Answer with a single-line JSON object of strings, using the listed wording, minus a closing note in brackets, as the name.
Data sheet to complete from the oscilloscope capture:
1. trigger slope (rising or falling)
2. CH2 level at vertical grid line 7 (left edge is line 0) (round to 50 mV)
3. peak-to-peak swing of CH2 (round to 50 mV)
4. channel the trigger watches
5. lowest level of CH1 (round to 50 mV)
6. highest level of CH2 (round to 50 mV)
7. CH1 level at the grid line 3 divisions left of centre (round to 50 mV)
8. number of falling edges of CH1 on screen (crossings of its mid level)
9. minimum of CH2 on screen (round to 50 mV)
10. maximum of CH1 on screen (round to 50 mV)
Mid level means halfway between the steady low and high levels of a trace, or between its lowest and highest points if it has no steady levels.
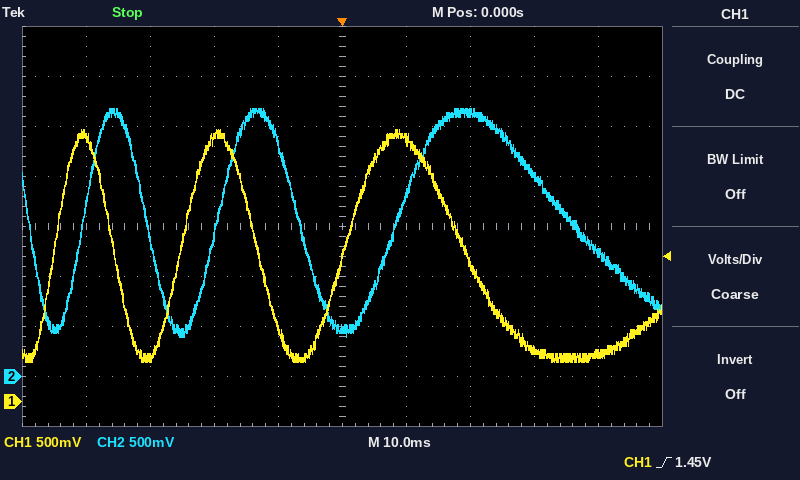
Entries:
{"trigger slope": "rising", "CH2 level at vertical grid line 7 (left edge is line 0)": "2.65 V", "peak-to-peak swing of CH2": "2.30 V", "channel the trigger watches": "CH1", "lowest level of CH1": "400 mV", "highest level of CH2": "2.70 V", "CH1 level at the grid line 3 divisions left of centre": "450 mV", "number of falling edges of CH1 on screen": "3", "minimum of CH2 on screen": "400 mV", "maximum of CH1 on screen": "2.70 V"}
